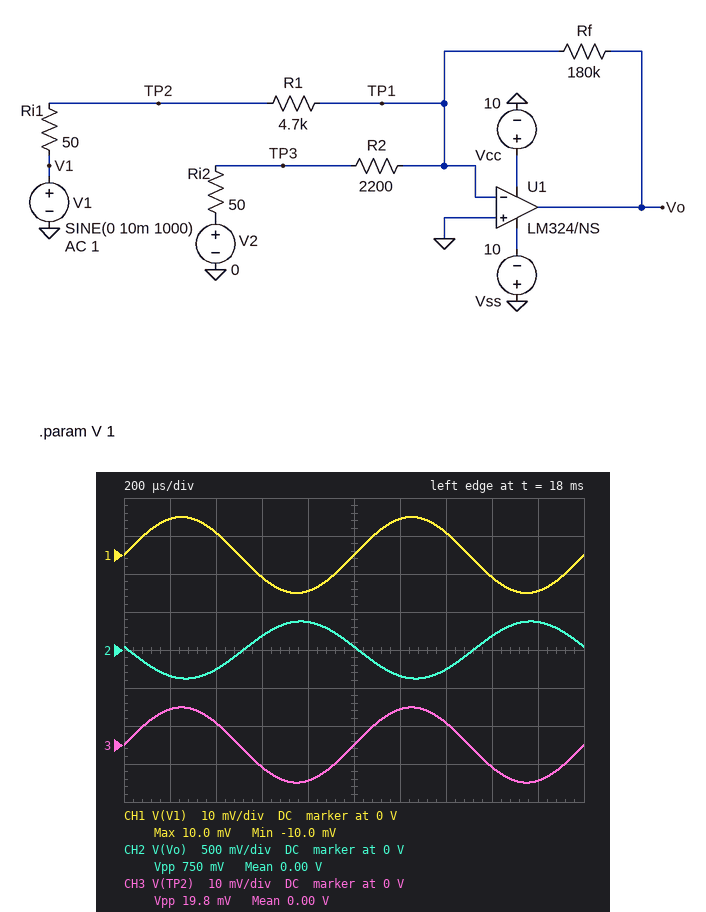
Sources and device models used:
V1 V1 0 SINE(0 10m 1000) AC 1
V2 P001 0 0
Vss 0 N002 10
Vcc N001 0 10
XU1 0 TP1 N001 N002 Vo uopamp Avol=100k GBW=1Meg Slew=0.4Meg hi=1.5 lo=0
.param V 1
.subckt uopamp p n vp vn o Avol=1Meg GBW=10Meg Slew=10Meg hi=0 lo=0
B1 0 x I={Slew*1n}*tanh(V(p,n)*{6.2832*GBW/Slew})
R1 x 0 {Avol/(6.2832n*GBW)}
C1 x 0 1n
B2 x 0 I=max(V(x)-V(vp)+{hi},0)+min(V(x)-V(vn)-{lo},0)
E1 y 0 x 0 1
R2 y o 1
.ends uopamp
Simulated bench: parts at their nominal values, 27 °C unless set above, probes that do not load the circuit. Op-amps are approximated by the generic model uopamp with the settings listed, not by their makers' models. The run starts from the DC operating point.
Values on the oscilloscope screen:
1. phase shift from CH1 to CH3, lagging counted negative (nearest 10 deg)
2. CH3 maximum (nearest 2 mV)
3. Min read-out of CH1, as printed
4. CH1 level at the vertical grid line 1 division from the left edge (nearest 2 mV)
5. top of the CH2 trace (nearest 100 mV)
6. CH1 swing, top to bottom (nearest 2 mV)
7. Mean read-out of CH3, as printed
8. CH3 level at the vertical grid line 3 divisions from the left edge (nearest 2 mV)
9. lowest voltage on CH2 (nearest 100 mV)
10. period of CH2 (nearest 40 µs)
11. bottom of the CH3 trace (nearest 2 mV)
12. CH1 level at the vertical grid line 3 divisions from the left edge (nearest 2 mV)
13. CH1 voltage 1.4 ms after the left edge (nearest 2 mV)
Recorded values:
0 deg
10 mV
-10.0 mV
10 mV
400 mV
20 mV
0.00 V
-6 mV
-400 mV
1.00 ms
-10 mV
-6 mV
6 mV
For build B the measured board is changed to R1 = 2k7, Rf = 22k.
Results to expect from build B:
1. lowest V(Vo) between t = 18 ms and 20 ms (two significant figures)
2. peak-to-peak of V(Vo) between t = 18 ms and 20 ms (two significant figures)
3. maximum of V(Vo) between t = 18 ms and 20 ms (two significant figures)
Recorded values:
-80 mV
160 mV
80 mV
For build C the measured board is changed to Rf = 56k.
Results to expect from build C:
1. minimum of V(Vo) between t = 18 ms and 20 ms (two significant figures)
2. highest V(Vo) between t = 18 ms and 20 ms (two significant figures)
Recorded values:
-120 mV
120 mV
